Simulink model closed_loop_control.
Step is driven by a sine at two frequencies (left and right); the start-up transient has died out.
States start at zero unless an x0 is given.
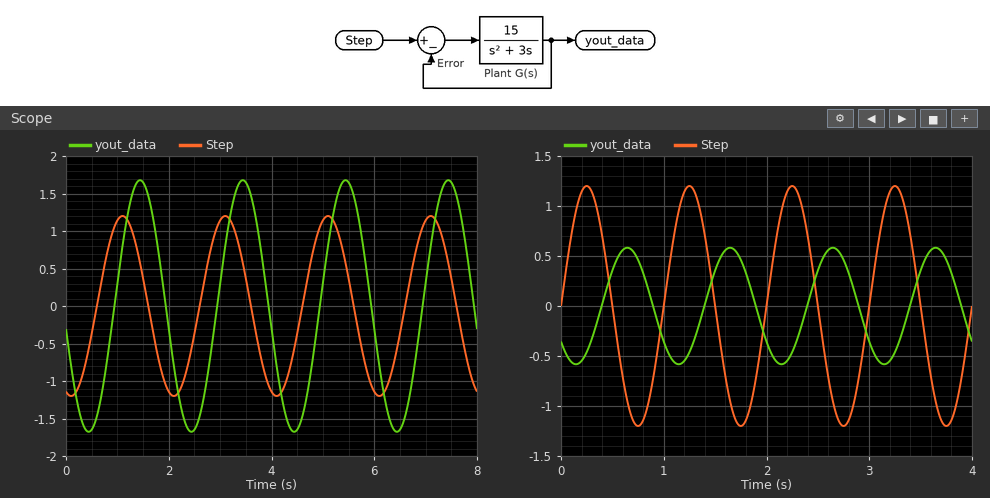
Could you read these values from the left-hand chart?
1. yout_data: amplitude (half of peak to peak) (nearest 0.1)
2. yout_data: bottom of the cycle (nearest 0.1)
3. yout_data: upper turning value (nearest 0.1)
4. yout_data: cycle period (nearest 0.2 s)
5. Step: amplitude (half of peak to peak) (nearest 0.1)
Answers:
1.7
-1.7
1.7
2.0 s
1.2
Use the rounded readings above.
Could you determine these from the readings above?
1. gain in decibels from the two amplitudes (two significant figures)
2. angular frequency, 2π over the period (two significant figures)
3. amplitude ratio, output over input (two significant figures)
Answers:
3.0 dB
3.1 rad/s
1.4
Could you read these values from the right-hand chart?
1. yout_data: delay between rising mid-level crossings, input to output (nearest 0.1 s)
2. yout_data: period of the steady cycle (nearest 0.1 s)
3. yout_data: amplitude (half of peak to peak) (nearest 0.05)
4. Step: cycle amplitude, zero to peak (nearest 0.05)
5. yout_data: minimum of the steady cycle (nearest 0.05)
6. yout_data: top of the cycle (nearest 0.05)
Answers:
0.4 s
1.0 s
0.60
1.20
-0.60
0.60
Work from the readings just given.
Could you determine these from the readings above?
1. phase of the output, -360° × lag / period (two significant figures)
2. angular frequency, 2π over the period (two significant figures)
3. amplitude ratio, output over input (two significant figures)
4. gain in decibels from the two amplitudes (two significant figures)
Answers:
-140°
6.3 rad/s
0.50
-6.0 dB
